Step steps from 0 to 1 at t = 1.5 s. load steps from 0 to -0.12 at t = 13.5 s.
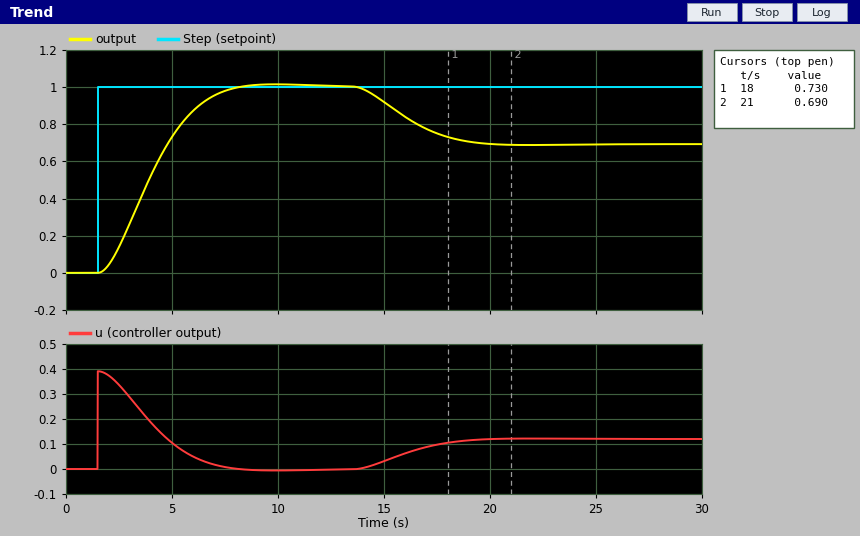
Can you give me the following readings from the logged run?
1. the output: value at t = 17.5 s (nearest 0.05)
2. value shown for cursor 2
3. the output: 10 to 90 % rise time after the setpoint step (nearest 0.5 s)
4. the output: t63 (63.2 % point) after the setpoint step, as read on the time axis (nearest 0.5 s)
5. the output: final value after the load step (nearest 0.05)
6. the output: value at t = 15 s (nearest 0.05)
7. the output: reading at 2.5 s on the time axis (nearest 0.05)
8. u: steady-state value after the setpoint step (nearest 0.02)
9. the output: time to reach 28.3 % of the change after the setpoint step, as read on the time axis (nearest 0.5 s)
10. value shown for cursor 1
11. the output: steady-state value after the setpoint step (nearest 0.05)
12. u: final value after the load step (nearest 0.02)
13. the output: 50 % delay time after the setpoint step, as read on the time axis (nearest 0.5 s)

0.75
0.690
4.0 s
4.5 s
0.70
0.90
0.15
0.00
3.0 s
0.730
1.00
0.12
4.0 s
